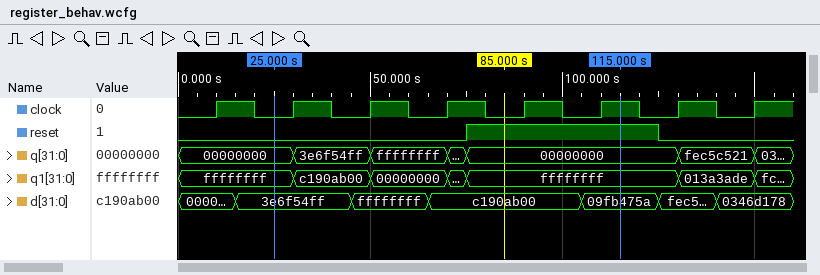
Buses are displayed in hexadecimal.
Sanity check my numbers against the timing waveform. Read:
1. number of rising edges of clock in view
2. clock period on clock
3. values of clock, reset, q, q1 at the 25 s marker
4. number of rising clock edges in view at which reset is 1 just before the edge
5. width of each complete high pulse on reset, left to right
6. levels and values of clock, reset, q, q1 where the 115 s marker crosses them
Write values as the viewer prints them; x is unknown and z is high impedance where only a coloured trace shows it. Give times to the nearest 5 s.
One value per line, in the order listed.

8
20 s
clock=0, reset=0, q=00000000, q1=ffffffff
2
50 s
clock=1, reset=1, q=00000000, q1=ffffffff
